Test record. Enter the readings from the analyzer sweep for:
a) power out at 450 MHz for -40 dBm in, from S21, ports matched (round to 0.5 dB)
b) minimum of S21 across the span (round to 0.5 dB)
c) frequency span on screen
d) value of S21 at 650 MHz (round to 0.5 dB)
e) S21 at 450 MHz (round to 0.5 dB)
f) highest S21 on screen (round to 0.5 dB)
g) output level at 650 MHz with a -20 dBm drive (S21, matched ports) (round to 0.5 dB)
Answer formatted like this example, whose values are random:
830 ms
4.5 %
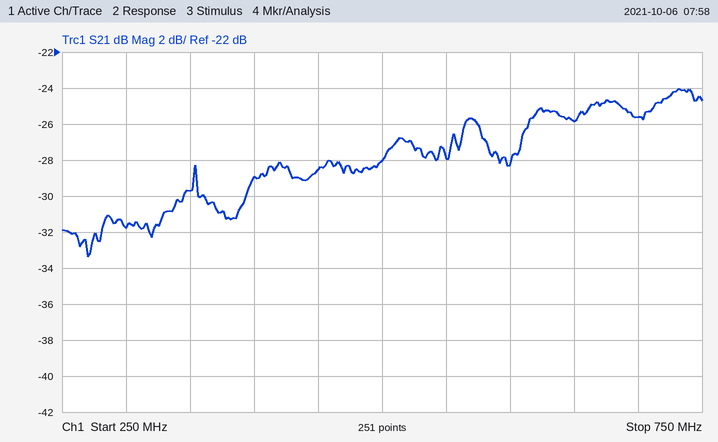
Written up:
-68.5 dBm
-33.5 dB
500 MHz
-26.0 dB
-28.5 dB
-24.0 dB
-46.0 dBm
